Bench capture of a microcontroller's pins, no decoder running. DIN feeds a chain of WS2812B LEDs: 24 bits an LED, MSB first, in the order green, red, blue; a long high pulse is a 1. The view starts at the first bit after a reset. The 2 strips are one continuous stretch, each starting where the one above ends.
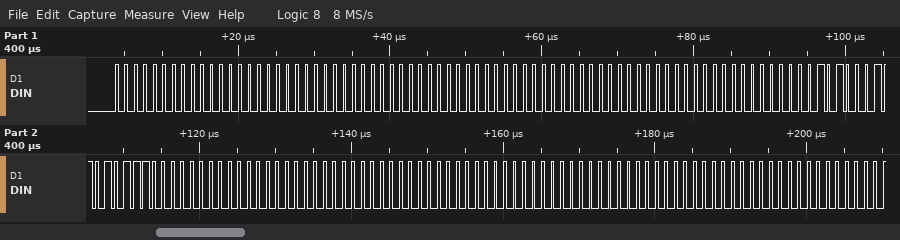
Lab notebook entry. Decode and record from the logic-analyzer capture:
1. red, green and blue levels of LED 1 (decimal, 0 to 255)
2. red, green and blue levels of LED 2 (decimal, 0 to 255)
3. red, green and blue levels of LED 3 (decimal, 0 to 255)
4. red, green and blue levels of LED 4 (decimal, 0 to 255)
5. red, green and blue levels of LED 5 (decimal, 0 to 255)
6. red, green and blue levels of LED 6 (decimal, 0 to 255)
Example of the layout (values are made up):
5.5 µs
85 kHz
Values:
0, 0, 0
0, 0, 0
0, 0, 0
215, 40, 0
0, 0, 0
0, 0, 0
